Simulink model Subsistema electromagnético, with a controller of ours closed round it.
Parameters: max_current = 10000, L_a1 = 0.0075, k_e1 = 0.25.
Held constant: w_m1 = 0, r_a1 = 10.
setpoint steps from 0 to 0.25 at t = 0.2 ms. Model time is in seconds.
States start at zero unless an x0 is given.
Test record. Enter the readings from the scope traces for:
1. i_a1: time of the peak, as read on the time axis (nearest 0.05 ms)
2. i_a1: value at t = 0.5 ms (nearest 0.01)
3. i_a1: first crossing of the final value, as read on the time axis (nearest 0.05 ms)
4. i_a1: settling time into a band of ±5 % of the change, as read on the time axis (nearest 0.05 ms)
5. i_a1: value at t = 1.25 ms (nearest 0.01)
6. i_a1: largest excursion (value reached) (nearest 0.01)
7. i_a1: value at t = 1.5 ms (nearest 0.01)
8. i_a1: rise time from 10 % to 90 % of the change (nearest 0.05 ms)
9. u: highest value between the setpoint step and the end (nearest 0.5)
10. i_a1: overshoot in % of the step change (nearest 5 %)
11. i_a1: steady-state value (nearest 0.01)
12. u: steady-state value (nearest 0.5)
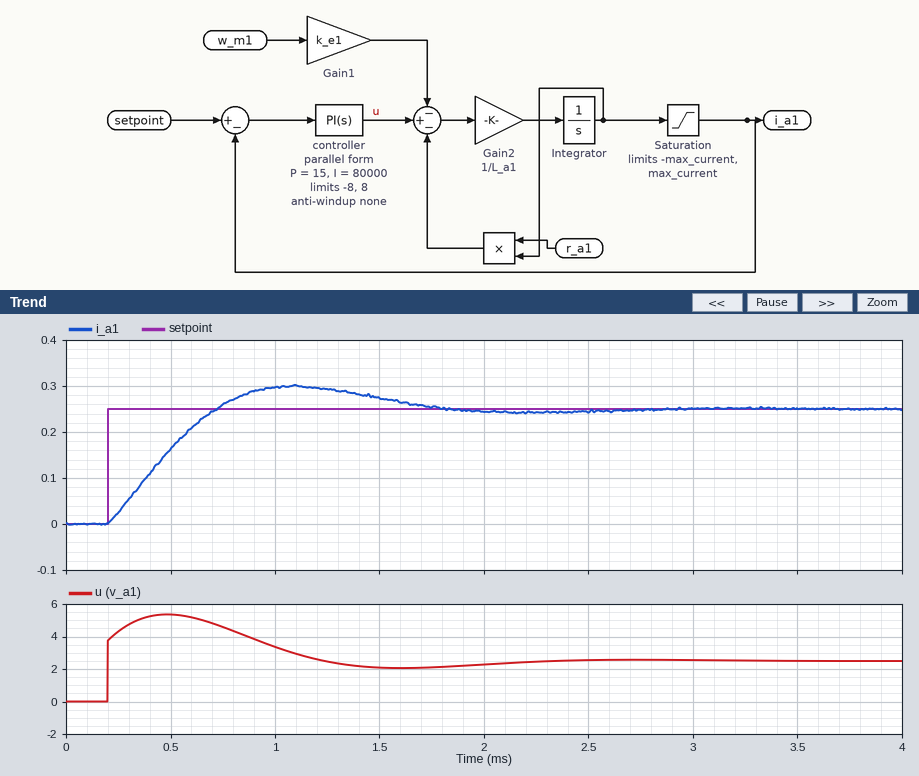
1.10 ms
0.16
0.70 ms
1.65 ms
0.29
0.30
0.27
0.40 ms
5.5
20 %
0.25
2.5
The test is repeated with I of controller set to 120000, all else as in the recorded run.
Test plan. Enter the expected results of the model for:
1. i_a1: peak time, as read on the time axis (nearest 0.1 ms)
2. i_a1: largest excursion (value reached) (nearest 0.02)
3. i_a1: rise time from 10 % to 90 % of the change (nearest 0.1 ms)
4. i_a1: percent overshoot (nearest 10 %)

0.9 ms
0.32
0.3 ms
30 %
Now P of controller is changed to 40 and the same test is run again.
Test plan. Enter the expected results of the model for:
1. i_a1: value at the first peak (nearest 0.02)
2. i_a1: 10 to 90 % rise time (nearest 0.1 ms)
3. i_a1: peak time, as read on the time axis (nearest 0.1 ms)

0.26
0.3 ms
1.0 ms
